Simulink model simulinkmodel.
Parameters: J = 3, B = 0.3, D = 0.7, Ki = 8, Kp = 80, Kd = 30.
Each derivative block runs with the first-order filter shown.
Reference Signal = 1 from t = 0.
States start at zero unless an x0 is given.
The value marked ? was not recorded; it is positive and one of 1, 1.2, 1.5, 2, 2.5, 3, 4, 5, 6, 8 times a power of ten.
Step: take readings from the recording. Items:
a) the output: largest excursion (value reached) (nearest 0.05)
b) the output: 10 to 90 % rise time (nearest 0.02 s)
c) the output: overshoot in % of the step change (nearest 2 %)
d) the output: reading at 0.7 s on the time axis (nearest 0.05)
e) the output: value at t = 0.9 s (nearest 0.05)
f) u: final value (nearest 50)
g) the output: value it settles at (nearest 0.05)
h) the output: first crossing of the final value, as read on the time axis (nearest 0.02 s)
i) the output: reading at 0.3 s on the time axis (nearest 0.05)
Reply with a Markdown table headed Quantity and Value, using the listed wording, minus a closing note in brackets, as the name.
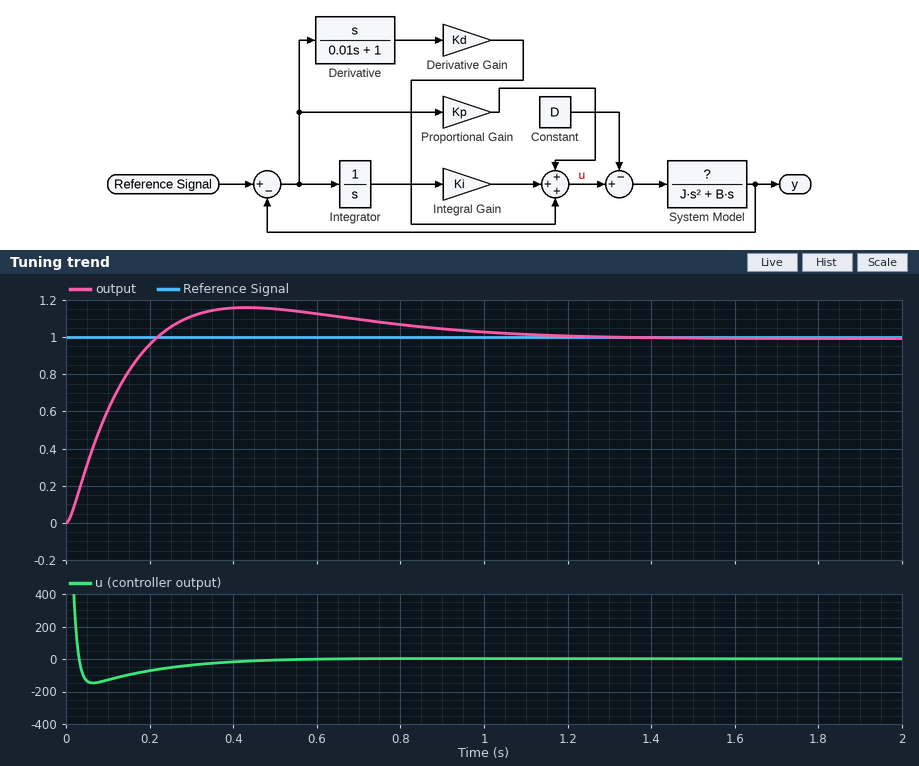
| Quantity | Value |
|---|---|
| the output: largest excursion (value reached) | 1.15 |
| the output: 10 to 90 % rise time | 0.16 s |
| the output: overshoot in % of the step change | 16 % |
| the output: reading at 0.7 s on the time axis | 1.10 |
| the output: value at t = 0.9 s | 1.05 |
| u: final value | 0 |
| the output: value it settles at | 1.00 |
| the output: first crossing of the final value, as read on the time axis | 0.22 s |
| the output: reading at 0.3 s on the time axis | 1.10 |
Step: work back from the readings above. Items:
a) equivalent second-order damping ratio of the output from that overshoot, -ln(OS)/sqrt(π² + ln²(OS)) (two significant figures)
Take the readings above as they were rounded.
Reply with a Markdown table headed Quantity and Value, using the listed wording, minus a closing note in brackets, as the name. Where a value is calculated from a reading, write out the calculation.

| Quantity | Value |
|---|---|
| equivalent second-order damping ratio of the output from that overshoot, -ln(OS)/sqrt(π² + ln²(OS)) | ln(0.16) = -1.833; 1.833 / sqrt(9.870 + 3.358) = 0.50 |
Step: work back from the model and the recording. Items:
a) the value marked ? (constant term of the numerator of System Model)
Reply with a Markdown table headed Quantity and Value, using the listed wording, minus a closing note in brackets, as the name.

| Quantity | Value |
|---|---|
| the value marked ? | 0.8 |
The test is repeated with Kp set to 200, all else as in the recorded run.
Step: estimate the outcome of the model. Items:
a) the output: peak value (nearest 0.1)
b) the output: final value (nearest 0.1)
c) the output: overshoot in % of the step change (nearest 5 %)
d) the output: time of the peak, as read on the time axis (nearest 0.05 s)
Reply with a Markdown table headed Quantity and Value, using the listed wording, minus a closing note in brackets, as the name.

| Quantity | Value |
|---|---|
| the output: peak value | 1.3 |
| the output: final value | 1.0 |
| the output: overshoot in % of the step change | 30 % |
| the output: time of the peak, as read on the time axis | 0.30 s |
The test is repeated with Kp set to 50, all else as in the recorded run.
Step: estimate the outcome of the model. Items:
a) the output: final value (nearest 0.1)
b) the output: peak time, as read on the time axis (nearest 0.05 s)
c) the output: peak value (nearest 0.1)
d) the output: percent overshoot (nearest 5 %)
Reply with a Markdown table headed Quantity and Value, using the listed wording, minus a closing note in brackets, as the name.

| Quantity | Value |
|---|---|
| the output: final value | 1.0 |
| the output: peak time, as read on the time axis | 0.50 s |
| the output: peak value | 1.1 |
| the output: percent overshoot | 10 % |
